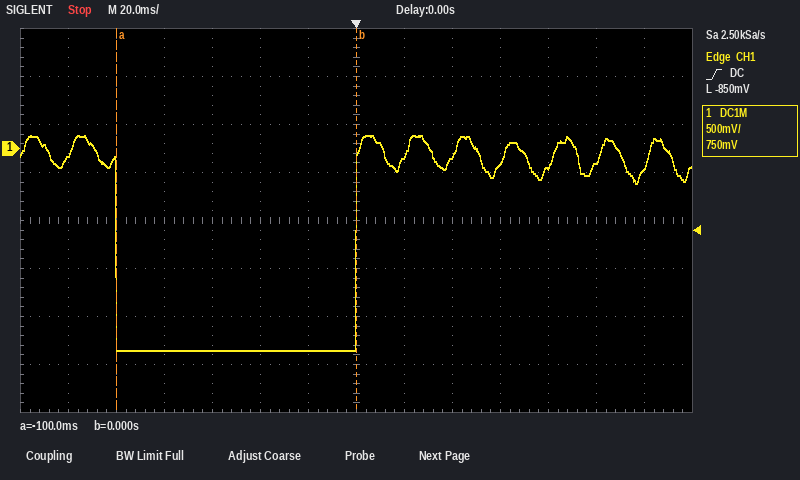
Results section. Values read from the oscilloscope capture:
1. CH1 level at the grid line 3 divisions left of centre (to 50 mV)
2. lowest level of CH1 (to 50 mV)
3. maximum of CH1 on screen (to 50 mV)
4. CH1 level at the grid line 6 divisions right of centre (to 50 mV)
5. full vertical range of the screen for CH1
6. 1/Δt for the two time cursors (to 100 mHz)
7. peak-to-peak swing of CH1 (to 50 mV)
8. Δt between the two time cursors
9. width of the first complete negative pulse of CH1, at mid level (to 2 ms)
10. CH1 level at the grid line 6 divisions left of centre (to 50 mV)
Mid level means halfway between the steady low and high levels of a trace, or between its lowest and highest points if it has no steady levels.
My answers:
-2.10 V
-2.10 V
150 mV
-200 mV
4 V
10.0 Hz
2.25 V
100 ms
100 ms
-100 mV
